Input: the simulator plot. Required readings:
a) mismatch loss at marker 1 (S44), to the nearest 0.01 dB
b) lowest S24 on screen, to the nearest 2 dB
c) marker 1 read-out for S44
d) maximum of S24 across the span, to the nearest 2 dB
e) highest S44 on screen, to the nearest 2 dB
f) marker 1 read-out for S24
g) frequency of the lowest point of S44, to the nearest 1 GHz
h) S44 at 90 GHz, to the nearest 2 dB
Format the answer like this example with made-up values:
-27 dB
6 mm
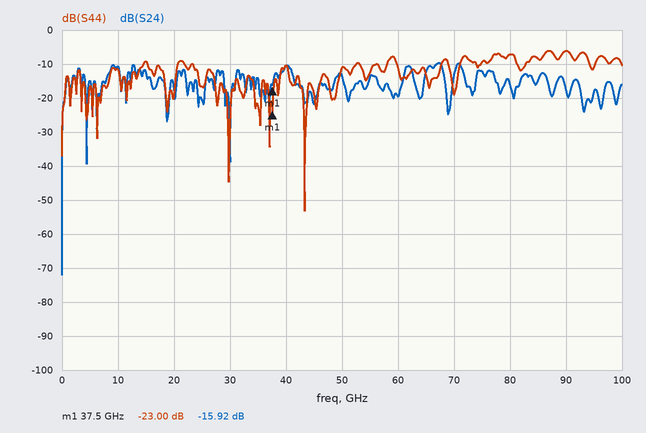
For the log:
0.02 dB
-72 dB
-23.00 dB
-10 dB
-6 dB
-15.92 dB
43 GHz
-6 dB
